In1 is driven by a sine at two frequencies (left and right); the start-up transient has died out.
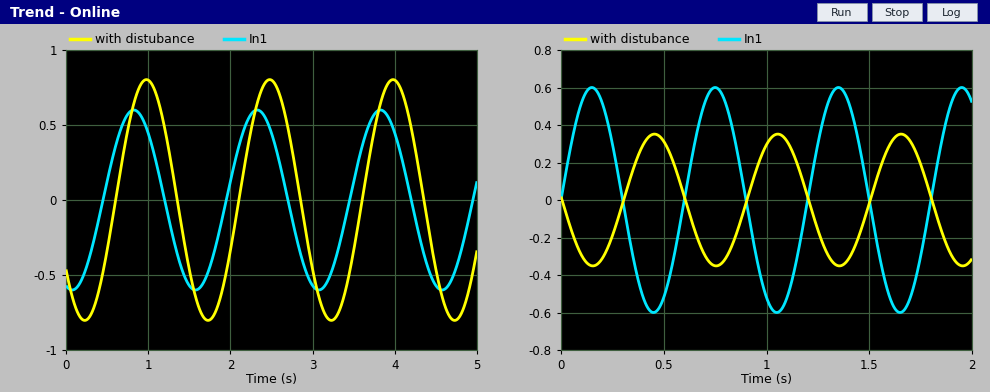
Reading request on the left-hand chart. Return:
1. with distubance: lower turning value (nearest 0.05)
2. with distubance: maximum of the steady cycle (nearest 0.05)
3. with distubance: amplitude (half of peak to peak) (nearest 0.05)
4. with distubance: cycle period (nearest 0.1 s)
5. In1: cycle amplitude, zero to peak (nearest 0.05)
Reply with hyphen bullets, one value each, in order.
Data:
- -0.80
- 0.80
- 0.80
- 1.5 s
- 0.60
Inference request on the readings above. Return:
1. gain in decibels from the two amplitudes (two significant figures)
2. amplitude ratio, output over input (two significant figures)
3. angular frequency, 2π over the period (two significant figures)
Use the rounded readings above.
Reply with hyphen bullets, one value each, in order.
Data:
- 2.5 dB
- 1.3
- 4.2 rad/s
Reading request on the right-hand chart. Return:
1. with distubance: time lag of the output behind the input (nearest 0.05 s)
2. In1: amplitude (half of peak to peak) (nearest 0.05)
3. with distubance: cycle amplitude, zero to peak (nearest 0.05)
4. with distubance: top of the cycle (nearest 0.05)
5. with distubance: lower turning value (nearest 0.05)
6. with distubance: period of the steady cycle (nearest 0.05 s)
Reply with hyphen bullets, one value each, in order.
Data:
- 0.30 s
- 0.60
- 0.35
- 0.35
- -0.35
- 0.60 s
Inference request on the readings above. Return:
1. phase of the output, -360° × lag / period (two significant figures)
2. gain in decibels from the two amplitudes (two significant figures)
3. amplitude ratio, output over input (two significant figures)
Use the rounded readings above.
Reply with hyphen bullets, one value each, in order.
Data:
- -180°
- -4.7 dB
- 0.58
